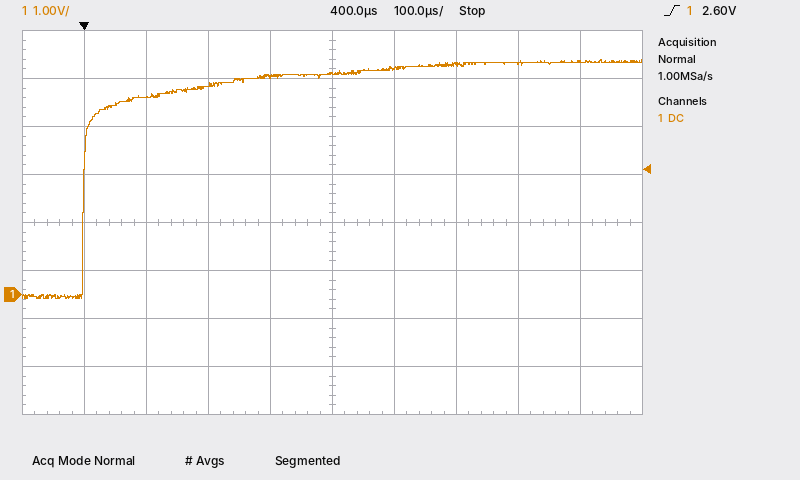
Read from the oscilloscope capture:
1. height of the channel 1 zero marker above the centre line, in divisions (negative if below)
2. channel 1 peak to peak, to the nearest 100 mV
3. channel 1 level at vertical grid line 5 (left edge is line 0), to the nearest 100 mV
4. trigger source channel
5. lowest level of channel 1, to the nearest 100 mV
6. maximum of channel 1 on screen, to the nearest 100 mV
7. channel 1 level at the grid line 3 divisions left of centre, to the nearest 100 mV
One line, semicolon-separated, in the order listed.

-1.5 div; 5.0 V; 4.6 V; channel 1; -100 mV; 4.9 V; 4.1 V
